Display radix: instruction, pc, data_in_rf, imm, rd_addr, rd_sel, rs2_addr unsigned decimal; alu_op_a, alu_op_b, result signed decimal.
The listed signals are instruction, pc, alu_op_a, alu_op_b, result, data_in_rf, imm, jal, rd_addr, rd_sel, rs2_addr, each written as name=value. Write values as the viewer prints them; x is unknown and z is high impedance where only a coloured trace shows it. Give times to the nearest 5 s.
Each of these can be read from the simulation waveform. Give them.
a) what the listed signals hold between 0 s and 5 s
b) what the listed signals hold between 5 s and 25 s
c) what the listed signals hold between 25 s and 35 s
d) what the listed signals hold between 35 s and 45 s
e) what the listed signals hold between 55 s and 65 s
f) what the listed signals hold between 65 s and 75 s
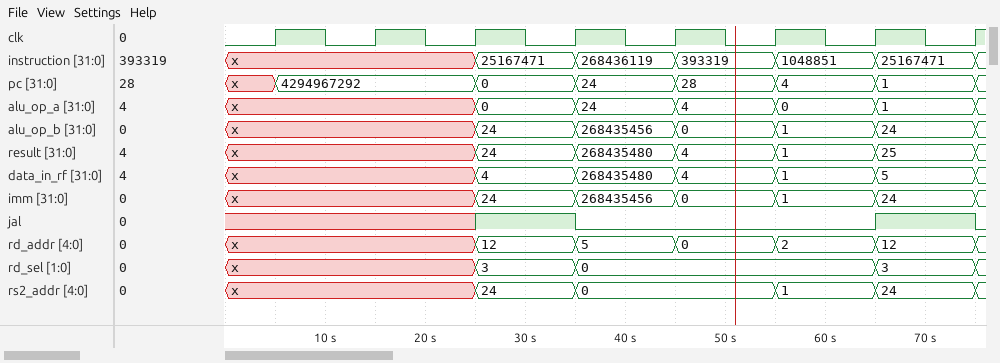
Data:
instruction=x, pc=x, alu_op_a=x, alu_op_b=x, result=x, data_in_rf=x, imm=x, jal=x, rd_addr=x, rd_sel=x, rs2_addr=x
instruction=x, pc=4294967292, alu_op_a=x, alu_op_b=x, result=x, data_in_rf=x, imm=x, jal=x, rd_addr=x, rd_sel=x, rs2_addr=x
instruction=25167471, pc=0, alu_op_a=0, alu_op_b=24, result=24, data_in_rf=4, imm=24, jal=1, rd_addr=12, rd_sel=3, rs2_addr=24
instruction=268436119, pc=24, alu_op_a=24, alu_op_b=268435456, result=268435480, data_in_rf=268435480, imm=268435456, jal=0, rd_addr=5, rd_sel=0, rs2_addr=0
instruction=1048851, pc=4, alu_op_a=0, alu_op_b=1, result=1, data_in_rf=1, imm=1, jal=0, rd_addr=2, rd_sel=0, rs2_addr=1
instruction=25167471, pc=1, alu_op_a=1, alu_op_b=24, result=25, data_in_rf=5, imm=24, jal=1, rd_addr=12, rd_sel=3, rs2_addr=24
